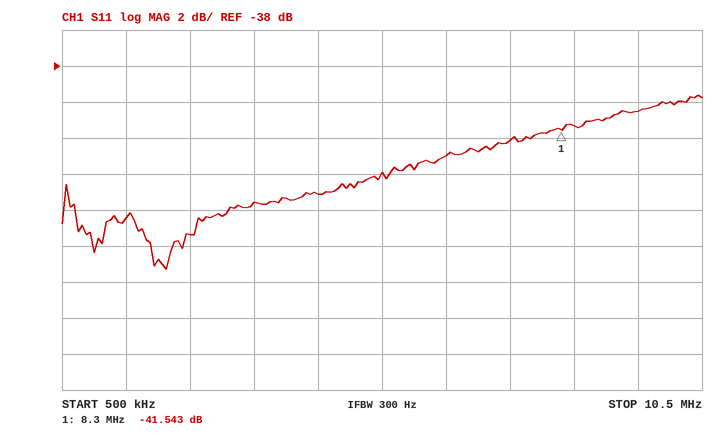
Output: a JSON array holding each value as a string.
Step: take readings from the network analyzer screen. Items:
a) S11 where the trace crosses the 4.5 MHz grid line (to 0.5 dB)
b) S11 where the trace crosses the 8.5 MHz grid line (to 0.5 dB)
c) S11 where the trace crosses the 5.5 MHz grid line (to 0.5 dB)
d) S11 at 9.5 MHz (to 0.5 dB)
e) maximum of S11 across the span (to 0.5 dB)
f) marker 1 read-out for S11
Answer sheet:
["-45.0 dB", "-41.5 dB", "-44.0 dB", "-40.5 dB", "-39.5 dB", "-41.543 dB"]
